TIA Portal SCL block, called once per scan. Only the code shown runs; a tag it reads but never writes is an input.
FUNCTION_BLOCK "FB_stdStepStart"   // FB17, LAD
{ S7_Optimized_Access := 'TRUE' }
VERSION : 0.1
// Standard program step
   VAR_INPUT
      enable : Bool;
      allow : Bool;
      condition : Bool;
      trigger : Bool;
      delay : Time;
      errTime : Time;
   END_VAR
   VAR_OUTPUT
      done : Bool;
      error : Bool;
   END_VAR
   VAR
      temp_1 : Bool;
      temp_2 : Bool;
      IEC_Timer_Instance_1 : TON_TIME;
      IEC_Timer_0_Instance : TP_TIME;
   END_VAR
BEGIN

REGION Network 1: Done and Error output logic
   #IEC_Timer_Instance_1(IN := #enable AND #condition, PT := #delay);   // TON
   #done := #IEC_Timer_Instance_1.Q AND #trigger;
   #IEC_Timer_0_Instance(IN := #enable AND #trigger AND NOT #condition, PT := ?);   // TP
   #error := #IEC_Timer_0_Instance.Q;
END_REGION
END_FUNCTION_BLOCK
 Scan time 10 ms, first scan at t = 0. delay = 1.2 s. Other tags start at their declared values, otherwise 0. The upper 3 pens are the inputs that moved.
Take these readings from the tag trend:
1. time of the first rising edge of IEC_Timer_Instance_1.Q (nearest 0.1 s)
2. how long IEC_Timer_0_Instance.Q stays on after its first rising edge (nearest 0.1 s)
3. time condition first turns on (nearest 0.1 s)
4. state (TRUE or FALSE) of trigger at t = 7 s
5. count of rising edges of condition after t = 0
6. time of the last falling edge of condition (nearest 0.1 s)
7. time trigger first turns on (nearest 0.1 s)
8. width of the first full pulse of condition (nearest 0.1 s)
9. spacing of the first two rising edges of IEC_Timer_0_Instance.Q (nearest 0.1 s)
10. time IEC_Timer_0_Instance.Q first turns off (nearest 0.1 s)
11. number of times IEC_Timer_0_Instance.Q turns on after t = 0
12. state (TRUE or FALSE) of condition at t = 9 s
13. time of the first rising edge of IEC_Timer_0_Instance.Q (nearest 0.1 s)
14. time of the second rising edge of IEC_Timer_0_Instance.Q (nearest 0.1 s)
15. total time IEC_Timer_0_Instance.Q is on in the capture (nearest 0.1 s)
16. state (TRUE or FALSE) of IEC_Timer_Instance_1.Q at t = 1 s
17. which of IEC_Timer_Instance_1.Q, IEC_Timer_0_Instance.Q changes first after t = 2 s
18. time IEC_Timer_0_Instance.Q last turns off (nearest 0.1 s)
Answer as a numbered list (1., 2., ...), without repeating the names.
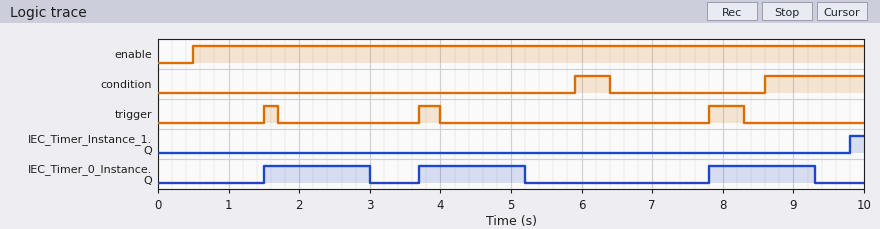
1. 9.8 s
2. 1.5 s
3. 5.9 s
4. FALSE
5. 2
6. 6.4 s
7. 1.5 s
8. 0.5 s
9. 2.2 s
10. 3.0 s
11. 3
12. TRUE
13. 1.5 s
14. 3.7 s
15. 4.5 s
16. FALSE
17. IEC_Timer_0_Instance.Q
18. 9.3 s
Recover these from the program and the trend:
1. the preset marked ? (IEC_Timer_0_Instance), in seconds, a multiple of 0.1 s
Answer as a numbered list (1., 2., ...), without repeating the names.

1. 1.5 s
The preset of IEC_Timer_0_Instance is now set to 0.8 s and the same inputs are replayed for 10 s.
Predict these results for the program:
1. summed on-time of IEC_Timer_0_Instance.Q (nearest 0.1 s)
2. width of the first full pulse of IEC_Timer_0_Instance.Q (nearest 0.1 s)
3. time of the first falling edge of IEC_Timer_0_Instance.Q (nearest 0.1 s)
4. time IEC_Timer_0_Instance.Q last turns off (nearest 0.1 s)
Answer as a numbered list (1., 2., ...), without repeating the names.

1. 2.4 s
2. 0.8 s
3. 2.3 s
4. 8.6 s
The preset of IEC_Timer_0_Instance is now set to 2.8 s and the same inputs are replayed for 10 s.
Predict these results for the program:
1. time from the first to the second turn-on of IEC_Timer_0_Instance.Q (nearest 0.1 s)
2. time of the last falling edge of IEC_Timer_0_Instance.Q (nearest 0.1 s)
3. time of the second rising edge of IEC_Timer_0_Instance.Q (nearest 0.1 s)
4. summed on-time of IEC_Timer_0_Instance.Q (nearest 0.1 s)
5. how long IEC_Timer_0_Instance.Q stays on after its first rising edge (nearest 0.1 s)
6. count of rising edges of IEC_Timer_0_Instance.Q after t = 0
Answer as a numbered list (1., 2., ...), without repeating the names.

1. 6.3 s
2. 4.3 s
3. 7.8 s
4. 5.0 s
5. 2.8 s
6. 2
